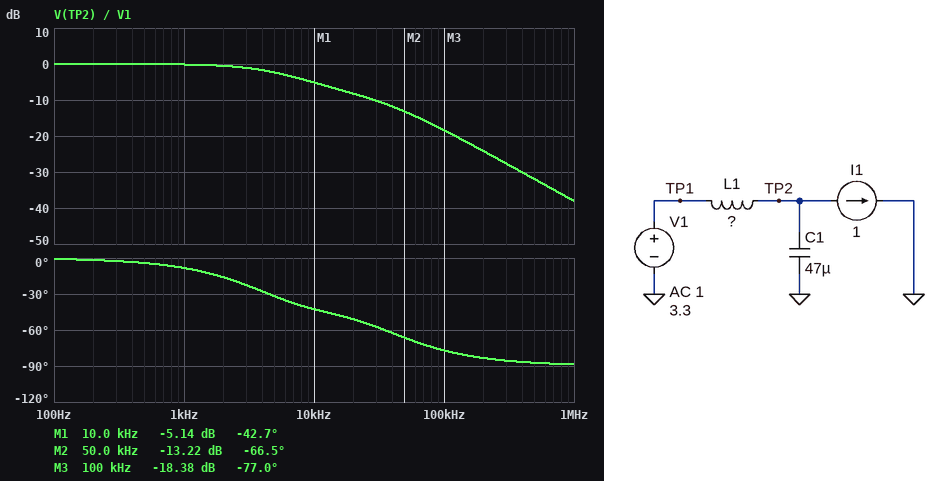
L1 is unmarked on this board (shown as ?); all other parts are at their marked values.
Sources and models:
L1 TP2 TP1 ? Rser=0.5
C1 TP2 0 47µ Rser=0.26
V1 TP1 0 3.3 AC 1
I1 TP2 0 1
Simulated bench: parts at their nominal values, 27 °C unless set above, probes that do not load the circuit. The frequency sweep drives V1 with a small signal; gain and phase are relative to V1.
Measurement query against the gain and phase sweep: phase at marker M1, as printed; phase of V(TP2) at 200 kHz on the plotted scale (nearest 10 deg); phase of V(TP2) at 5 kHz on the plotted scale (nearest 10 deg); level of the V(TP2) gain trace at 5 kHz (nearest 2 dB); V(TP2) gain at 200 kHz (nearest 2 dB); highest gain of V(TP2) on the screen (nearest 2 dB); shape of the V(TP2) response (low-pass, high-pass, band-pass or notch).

-42.7 deg
-80 deg
-30 deg
-2 dB
-24 dB
0 dB
low-pass
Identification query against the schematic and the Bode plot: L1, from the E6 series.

3.3 µH
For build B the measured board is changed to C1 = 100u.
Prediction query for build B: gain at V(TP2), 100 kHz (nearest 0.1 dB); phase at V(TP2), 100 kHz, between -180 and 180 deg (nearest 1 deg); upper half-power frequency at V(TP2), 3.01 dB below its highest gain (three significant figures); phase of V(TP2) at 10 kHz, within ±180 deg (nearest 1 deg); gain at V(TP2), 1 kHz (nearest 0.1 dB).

-18.5 dB
-73 deg
2.58 kHz
-35 deg
-0.7 dB
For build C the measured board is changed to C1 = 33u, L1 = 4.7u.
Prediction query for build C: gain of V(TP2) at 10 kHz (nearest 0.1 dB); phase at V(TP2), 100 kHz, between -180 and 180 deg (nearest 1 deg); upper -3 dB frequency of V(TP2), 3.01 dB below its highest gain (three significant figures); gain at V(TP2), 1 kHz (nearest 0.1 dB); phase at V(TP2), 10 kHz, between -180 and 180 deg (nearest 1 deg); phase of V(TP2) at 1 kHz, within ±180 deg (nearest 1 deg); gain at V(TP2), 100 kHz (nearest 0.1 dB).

-3.1 dB
-86 deg
9.81 kHz
0 dB
-48 deg
-6 deg
-21.1 dB
